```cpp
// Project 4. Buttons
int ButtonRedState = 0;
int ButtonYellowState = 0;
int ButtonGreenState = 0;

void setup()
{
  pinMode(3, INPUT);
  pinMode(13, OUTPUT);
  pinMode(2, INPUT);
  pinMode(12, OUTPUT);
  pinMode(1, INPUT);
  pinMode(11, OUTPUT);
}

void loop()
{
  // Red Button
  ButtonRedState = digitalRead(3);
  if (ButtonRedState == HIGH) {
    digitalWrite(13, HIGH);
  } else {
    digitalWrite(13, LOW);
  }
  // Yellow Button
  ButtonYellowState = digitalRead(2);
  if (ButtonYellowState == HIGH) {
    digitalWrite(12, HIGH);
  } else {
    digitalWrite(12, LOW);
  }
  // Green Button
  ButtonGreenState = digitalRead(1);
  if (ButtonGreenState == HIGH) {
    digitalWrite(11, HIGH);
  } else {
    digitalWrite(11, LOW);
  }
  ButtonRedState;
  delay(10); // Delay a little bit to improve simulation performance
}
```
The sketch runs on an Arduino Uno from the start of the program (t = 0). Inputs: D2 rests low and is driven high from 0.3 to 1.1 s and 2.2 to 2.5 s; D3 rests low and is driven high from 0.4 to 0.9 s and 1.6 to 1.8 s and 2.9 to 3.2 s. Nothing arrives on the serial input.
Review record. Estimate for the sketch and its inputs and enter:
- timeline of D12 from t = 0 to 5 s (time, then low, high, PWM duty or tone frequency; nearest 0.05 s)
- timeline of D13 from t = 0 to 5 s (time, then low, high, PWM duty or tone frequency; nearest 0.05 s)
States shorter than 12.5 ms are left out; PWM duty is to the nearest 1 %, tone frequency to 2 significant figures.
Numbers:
0 s low; 0.3 s high; 1.1 s low; 2.2 s high; 2.5 s low
0 s low; 0.4 s high; 0.9 s low; 1.6 s high; 1.8 s low; 2.9 s high; 3.2 s low
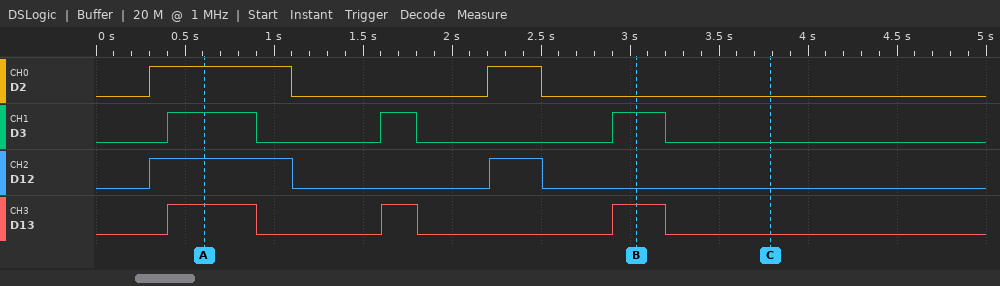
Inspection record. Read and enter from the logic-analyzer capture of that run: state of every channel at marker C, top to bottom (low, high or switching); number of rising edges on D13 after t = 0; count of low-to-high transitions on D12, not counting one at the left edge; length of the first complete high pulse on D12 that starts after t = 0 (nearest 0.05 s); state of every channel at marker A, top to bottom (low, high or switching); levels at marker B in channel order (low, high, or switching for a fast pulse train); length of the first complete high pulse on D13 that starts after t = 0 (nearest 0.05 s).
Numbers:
D2 low, D3 low, D12 low, D13 low
3
2
0.80 s
D2 high, D3 high, D12 high, D13 high
D2 low, D3 high, D12 low, D13 high
0.50 s
